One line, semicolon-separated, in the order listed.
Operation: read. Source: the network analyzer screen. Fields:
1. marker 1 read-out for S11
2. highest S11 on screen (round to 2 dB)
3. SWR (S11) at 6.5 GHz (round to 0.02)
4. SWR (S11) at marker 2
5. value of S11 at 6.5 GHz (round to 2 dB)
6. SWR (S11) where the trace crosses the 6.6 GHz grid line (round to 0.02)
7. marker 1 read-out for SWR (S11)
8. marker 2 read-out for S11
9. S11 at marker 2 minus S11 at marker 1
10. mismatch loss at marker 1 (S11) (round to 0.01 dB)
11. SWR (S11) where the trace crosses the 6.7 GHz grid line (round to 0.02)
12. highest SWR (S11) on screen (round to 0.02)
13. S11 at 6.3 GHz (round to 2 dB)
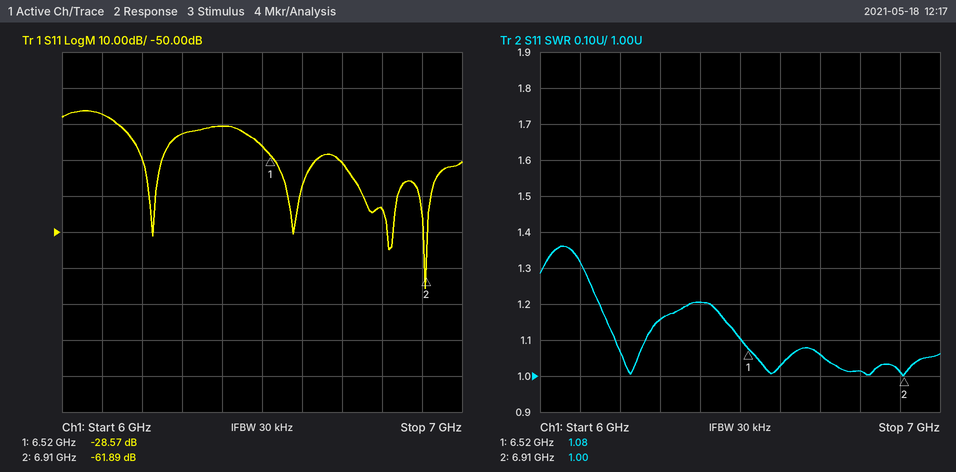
-28.57 dB; -16 dB; 1.10; 1.00; -26 dB; 1.02; 1.08; -61.89 dB; -33.32 dB; 0.01 dB; 1.06; 1.36; -22 dB
